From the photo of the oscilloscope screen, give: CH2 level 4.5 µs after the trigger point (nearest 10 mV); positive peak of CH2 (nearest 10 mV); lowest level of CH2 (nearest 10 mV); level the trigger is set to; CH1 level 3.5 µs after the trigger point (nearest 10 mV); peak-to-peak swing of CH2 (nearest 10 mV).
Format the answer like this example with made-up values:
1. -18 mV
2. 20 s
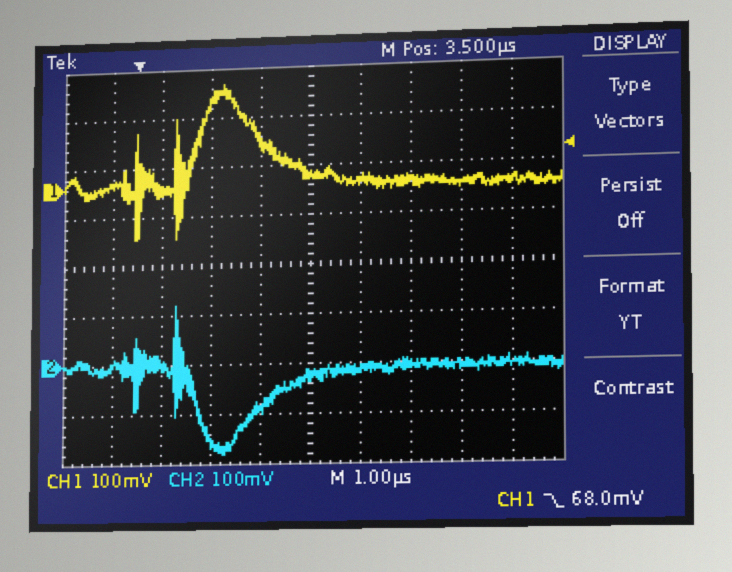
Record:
1. -10 mV
2. 120 mV
3. -180 mV
4. 68.0 mV
5. 20 mV
6. 300 mV
